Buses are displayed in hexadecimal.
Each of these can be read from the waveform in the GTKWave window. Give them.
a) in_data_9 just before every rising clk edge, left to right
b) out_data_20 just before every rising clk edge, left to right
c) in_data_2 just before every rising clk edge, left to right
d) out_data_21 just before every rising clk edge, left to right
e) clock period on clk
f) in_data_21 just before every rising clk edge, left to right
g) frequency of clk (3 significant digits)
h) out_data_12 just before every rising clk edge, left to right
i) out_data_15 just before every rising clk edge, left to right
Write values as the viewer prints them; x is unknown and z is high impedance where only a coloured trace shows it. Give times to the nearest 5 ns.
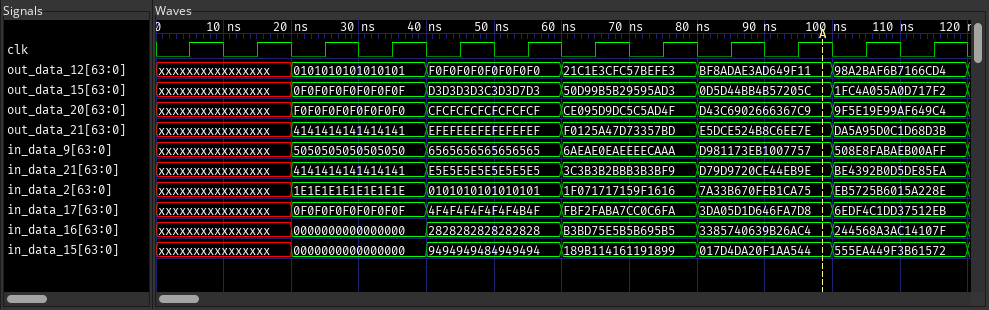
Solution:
xxxxxxxxxxxxxxxx, xxxxxxxxxxxxxxxx, 5050505050505050, 5050505050505050, 6565656565656565, 6565656565656565, 6AEAE0EAEEEECAAA, 6AEAE0EAEEEECAAA, D981173EB1007757, D981173EB1007757, 508E8FABAEB00AFF, 508E8FABAEB00AFF
xxxxxxxxxxxxxxxx, xxxxxxxxxxxxxxxx, F0F0F0F0F0F0F0F0, F0F0F0F0F0F0F0F0, CFCFCFCFCFCFCFCF, CFCFCFCFCFCFCFCF, CE095D9DC5C5AD4F, CE095D9DC5C5AD4F, D43C6902666367C9, D43C6902666367C9, 9F5E19E99AF649C4, 9F5E19E99AF649C4
xxxxxxxxxxxxxxxx, xxxxxxxxxxxxxxxx, 1E1E1E1E1E1E1E1E, 1E1E1E1E1E1E1E1E, 0101010101010101, 0101010101010101, 1F071717159F1616, 1F071717159F1616, 7A33B670FEB1CA75, 7A33B670FEB1CA75, EB5725B6015A228E, EB5725B6015A228E
xxxxxxxxxxxxxxxx, xxxxxxxxxxxxxxxx, 4141414141414141, 4141414141414141, EFEFEEEFEFEFEFEF, EFEFEEEFEFEFEFEF, F0125A47D73357BD, F0125A47D73357BD, E5DCE524B8C6EE7E, E5DCE524B8C6EE7E, DA5A95D0C1D68D3B, DA5A95D0C1D68D3B
10 ns
xxxxxxxxxxxxxxxx, xxxxxxxxxxxxxxxx, 4141414141414141, 4141414141414141, E5E5E5E5E5E5E5E5, E5E5E5E5E5E5E5E5, 3C3B3B2BBB3B3BF9, 3C3B3B2BBB3B3BF9, D79D9720CE44EB9E, D79D9720CE44EB9E, BE4392B0D5DE85EA, BE4392B0D5DE85EA
100 MHz
xxxxxxxxxxxxxxxx, xxxxxxxxxxxxxxxx, 0101010101010101, 0101010101010101, F0F0F0F0F0F0F0F0, F0F0F0F0F0F0F0F0, 21C1E3CFC57BEFE3, 21C1E3CFC57BEFE3, BF8ADAE3AD649F11, BF8ADAE3AD649F11, 98A2BAF6B7166CD4, 98A2BAF6B7166CD4
xxxxxxxxxxxxxxxx, xxxxxxxxxxxxxxxx, 0F0F0F0F0F0F0F0F, 0F0F0F0F0F0F0F0F, D3D3D3D3C3D3D7D3, D3D3D3D3C3D3D7D3, 50D99B5B29595AD3, 50D99B5B29595AD3, 0D5D44BB4B57205C, 0D5D44BB4B57205C, 1FC4A055A0D717F2, 1FC4A055A0D717F2
